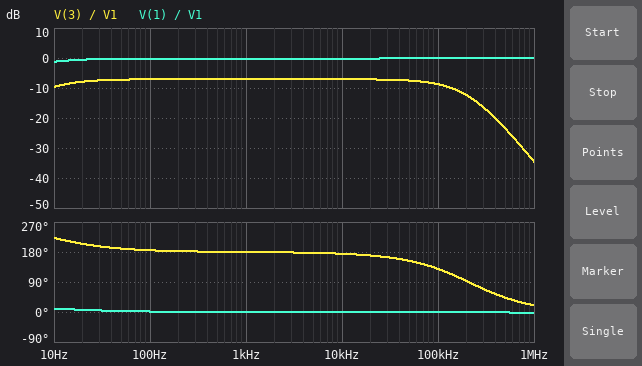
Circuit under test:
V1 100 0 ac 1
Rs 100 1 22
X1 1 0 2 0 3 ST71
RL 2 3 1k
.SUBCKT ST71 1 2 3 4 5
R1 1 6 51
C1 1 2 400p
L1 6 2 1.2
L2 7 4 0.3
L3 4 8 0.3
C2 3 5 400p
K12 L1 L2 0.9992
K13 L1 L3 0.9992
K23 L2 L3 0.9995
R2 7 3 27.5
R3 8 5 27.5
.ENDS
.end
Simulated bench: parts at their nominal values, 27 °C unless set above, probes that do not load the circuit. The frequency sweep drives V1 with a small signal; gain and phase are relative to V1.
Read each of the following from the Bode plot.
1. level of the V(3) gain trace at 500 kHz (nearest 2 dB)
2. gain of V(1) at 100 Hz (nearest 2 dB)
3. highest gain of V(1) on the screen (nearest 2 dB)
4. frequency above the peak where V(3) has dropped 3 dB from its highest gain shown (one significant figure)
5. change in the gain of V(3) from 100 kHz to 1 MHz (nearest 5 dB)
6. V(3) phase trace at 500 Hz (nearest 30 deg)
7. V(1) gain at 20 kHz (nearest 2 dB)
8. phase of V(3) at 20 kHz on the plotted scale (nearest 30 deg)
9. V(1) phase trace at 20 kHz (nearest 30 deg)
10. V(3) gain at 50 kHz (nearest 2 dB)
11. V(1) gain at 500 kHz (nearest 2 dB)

-24 dB
0 dB
0 dB
100 kHz
-25 dB
180 deg
0 dB
180 deg
0 deg
-8 dB
0 dB
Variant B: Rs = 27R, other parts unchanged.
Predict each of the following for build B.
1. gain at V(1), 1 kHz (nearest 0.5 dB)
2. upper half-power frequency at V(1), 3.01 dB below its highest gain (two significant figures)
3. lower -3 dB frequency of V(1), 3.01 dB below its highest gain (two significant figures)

0 dB
15 MHz
3.8 Hz
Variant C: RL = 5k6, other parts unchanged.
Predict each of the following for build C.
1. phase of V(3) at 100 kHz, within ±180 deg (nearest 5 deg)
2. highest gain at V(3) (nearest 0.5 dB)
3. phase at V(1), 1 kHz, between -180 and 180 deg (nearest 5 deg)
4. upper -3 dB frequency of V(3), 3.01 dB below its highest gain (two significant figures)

165 deg
1.5 dB
0 deg
230 kHz
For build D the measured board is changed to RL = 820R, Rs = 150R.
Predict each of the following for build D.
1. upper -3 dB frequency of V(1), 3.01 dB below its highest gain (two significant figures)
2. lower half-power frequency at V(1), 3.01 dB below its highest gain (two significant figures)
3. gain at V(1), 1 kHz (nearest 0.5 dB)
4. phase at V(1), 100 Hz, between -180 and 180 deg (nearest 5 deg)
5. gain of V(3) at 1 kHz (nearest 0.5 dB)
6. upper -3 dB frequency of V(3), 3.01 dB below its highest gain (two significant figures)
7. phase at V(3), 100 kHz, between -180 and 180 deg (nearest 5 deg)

2.7 MHz
28 Hz
-1.5 dB
10 deg
-8.5 dB
120 kHz
125 deg
